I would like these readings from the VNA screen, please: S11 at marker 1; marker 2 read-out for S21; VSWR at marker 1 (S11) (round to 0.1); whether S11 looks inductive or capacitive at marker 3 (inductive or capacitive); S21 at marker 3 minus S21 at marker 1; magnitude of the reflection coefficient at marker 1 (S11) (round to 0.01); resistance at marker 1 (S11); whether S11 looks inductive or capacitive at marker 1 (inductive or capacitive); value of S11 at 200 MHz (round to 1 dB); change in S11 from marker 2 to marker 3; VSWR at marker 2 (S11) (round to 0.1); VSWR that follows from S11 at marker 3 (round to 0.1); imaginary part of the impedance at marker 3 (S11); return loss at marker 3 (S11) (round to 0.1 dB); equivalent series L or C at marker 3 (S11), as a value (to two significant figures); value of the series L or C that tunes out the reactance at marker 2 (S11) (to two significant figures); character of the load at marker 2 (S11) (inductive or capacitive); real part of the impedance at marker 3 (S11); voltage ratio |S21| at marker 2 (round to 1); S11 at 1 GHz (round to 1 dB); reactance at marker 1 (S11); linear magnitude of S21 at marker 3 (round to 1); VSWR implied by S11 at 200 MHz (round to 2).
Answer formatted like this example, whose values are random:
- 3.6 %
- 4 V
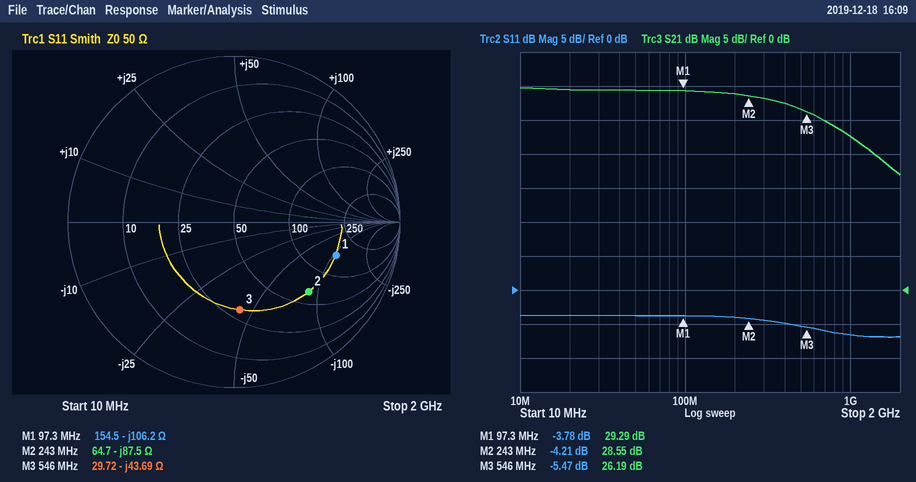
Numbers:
- -3.78 dB
- 28.55 dB
- 4.7
- capacitive
- -3.10 dB
- 0.65
- 154.5 Ω
- capacitive
- -4 dB
- -1.26 dB
- 4.2
- 3.3
- -43.69 Ω
- 5.5 dB
- 6.7 pF
- 57 nH
- capacitive
- 29.72 Ω
- 27
- -7 dB
- -106.2 Ω
- 20
- 4
